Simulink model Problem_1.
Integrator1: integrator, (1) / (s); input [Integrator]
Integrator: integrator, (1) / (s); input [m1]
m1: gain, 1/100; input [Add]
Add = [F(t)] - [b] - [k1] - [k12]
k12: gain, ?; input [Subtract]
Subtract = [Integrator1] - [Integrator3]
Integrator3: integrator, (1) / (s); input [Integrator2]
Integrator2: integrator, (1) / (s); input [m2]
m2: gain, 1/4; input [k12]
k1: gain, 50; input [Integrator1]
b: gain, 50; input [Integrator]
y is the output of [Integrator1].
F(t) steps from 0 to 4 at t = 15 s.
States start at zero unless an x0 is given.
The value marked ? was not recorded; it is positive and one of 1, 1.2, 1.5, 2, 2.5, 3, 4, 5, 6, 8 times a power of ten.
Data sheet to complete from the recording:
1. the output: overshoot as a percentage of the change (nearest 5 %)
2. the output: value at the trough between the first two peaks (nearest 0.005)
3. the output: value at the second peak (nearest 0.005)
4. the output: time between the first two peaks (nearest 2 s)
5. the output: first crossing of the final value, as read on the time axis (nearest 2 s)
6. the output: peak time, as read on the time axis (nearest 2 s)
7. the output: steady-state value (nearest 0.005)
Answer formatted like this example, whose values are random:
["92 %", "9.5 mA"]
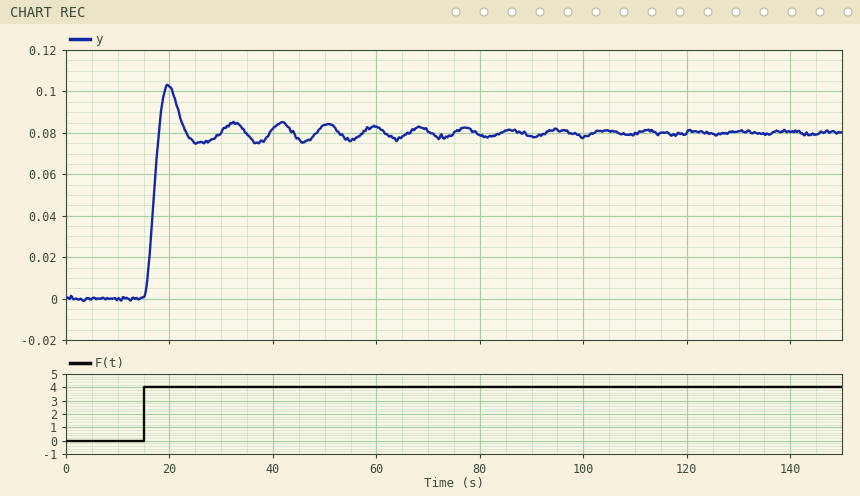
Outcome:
["30 %", "0.075", "0.085", "12 s", "18 s", "20 s", "0.080"]
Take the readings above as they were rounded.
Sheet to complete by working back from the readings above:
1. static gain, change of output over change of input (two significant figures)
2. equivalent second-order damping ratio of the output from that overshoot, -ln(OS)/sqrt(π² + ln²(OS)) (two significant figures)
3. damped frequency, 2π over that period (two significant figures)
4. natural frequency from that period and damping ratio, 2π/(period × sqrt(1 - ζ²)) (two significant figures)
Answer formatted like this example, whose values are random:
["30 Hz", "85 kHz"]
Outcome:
["0.020", "0.36", "0.52 rad/s", "0.56 rad/s"]
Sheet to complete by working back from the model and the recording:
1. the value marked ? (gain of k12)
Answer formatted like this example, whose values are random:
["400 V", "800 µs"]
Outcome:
["2"]
